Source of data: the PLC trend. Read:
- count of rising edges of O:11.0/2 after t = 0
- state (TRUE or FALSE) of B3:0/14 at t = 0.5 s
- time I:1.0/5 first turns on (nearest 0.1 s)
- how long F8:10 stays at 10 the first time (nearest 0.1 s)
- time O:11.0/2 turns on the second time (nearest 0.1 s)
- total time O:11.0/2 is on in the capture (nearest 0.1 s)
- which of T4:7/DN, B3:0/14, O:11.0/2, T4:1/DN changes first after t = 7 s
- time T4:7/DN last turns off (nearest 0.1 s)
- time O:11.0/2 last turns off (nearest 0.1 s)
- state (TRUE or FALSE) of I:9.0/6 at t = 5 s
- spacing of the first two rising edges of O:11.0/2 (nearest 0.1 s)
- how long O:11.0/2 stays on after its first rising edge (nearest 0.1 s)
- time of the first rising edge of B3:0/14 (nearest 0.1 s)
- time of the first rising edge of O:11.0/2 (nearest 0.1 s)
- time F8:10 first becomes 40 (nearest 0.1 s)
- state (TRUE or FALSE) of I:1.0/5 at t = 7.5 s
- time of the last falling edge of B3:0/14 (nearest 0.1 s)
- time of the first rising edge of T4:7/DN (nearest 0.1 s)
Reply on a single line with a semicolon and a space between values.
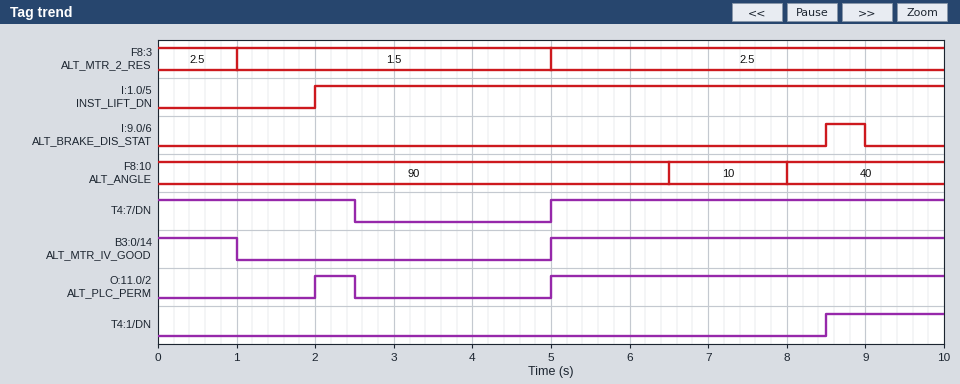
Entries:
2; TRUE; 2.0 s; 1.5 s; 5.0 s; 5.5 s; T4:1/DN; 2.5 s; 2.5 s; FALSE; 3.0 s; 0.5 s; 5.0 s; 2.0 s; 8.0 s; TRUE; 1.0 s; 5.0 s
